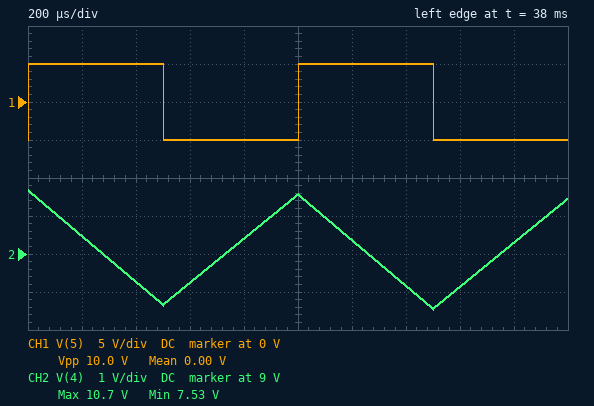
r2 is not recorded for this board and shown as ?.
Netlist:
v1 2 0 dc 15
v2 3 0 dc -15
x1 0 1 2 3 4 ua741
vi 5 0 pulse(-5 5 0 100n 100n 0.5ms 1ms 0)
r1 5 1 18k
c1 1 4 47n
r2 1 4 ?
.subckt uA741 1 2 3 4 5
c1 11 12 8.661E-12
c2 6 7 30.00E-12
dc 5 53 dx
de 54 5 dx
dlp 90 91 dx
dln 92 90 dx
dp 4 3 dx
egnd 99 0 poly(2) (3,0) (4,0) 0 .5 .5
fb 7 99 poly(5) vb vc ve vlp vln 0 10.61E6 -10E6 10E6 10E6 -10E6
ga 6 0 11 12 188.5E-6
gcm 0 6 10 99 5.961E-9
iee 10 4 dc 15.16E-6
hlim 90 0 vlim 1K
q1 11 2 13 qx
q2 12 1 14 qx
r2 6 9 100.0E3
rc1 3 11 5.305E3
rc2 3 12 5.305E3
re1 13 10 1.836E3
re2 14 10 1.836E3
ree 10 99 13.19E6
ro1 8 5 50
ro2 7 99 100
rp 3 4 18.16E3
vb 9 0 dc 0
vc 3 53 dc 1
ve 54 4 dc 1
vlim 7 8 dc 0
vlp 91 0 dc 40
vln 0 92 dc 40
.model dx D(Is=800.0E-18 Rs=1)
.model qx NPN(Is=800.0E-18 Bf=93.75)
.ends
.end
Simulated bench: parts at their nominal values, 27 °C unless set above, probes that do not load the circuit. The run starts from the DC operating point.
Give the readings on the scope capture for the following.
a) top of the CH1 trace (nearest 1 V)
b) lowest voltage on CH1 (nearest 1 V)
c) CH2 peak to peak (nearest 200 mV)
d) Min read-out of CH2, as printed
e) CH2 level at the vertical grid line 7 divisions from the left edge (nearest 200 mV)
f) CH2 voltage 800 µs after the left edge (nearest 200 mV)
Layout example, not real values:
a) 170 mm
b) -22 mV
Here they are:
a) 5 V
b) -5 V
c) 3.2 V
d) 7.53 V
e) 8.2 V
f) 9.4 V
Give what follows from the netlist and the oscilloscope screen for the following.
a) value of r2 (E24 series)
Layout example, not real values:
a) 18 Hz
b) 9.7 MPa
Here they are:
a) 1.8 MΩ
